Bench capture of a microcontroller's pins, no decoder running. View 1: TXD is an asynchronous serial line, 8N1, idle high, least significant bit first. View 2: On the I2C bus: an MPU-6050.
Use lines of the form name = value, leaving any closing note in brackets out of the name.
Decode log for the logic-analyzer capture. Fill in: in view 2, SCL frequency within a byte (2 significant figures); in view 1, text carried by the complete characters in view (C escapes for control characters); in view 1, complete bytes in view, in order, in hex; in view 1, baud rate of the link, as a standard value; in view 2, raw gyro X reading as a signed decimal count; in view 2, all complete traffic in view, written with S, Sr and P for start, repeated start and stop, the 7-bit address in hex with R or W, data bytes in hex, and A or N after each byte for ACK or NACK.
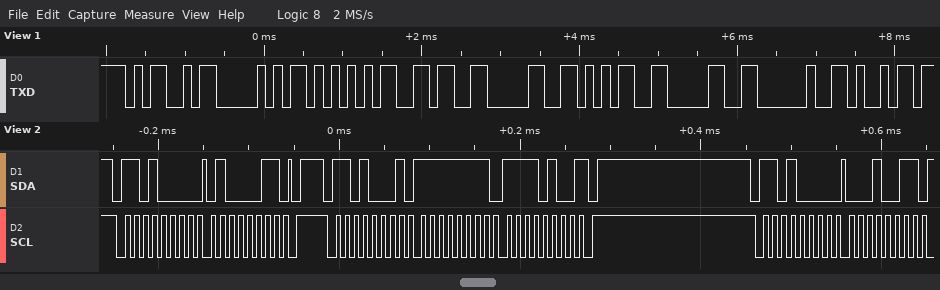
in view 2, SCL frequency within a byte = 100 kHz
in view 1, text carried by the complete characters in view = "MPU6050 i"
in view 1, complete bytes in view, in order, in hex = 4D 50 55 36 30 35 30 20 69
in view 1, baud rate of the link, as a standard value = 9600 baud
in view 2, raw gyro X reading as a signed decimal count = -12
in view 2, all complete traffic in view, written with S, Sr and P for start, repeated start and stop, the 7-bit address in hex with R or W, data bytes in hex, and A or N after each byte for ACK or NACK = S 68W A 43 A P S 68R A FF A F4 N P S 68W A 13 A
